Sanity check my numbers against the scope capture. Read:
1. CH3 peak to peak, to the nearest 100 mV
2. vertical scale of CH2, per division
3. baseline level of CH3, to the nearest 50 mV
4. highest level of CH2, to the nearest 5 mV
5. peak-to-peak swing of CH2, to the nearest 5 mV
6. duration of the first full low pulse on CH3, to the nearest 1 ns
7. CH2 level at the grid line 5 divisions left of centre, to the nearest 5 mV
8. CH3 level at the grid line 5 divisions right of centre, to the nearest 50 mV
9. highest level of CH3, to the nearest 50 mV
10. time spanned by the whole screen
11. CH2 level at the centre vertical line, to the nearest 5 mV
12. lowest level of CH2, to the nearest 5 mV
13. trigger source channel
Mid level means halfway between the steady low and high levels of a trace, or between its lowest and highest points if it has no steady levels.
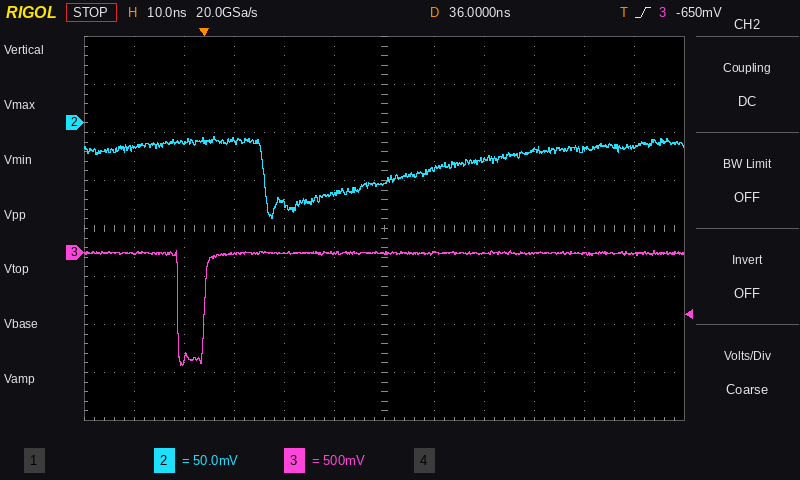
1.20 V
50 mV
0 mV
-15 mV
85 mV
5 ns
-25 mV
0 mV
0 mV
120 ns
-65 mV
-100 mV
CH3
